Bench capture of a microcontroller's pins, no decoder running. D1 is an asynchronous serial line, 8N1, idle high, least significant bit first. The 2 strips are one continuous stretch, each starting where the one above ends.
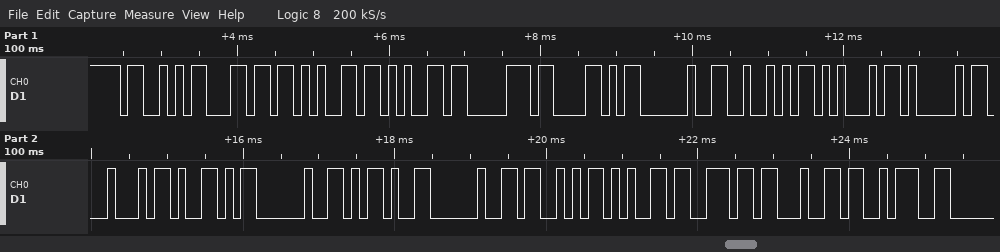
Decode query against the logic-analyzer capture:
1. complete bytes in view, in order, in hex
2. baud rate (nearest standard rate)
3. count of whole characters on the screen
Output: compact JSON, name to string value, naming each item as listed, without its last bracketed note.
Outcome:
{"complete bytes in view, in order, in hex": "53 6C 65 65 70 58 20 52 45 41 44 59 20 2D 20 53 65 6E 64 3A", "baud rate": "9600 baud", "count of whole characters on the screen": "20"}
